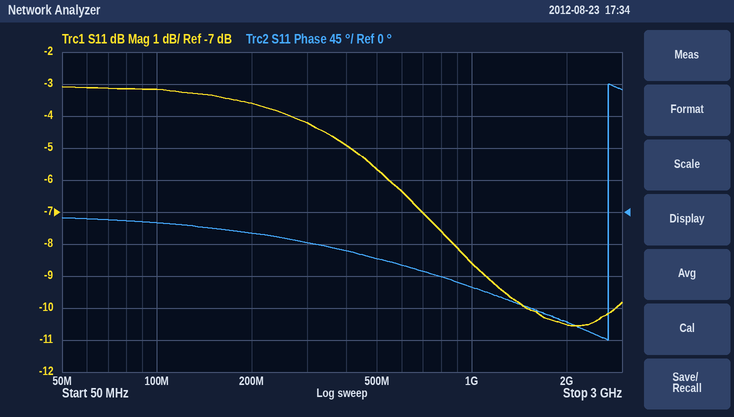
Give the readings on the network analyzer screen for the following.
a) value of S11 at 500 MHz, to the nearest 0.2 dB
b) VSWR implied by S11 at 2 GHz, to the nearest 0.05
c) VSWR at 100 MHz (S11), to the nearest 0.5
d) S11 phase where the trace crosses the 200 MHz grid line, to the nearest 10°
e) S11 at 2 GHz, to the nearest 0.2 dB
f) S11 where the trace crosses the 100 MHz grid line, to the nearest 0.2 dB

-5.6 dB
1.85
5.5
-30°
-10.6 dB
-3.2 dB
